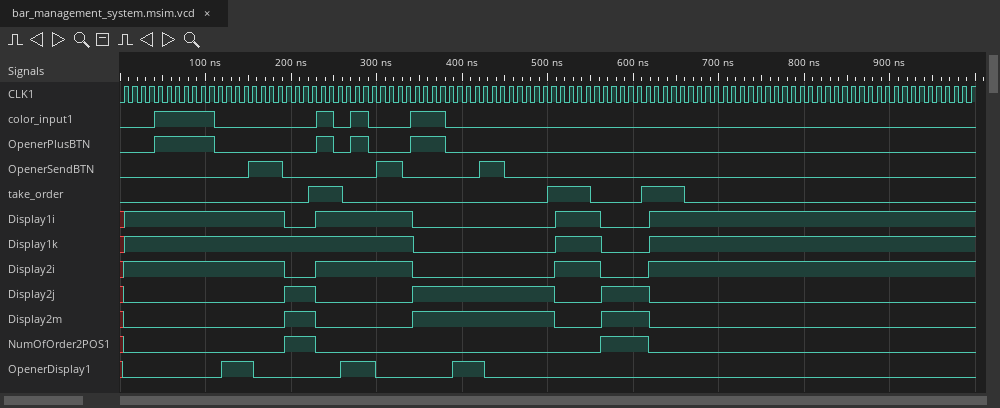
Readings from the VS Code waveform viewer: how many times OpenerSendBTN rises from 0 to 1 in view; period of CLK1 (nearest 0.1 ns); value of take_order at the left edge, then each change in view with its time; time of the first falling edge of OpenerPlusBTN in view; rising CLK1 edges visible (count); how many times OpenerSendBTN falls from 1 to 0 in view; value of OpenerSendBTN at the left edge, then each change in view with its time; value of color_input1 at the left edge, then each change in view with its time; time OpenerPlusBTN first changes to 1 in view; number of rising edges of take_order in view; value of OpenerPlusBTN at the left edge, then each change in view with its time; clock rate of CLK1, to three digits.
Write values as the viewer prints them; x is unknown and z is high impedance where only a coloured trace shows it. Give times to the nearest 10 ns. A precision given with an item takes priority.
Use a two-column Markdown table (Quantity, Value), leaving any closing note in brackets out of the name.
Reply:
| Quantity | Value |
|---|---|
| how many times OpenerSendBTN rises from 0 to 1 in view | 3 |
| period of CLK1 | 10 ns |
| value of take_order at the left edge, then each change in view with its time | 0, 1 at 220 ns, 0 at 260 ns, 1 at 500 ns, 0 at 550 ns, 1 at 610 ns, 0 at 660 ns |
| time of the first falling edge of OpenerPlusBTN in view | 110 ns |
| rising CLK1 edges visible | 100 |
| how many times OpenerSendBTN falls from 1 to 0 in view | 3 |
| value of OpenerSendBTN at the left edge, then each change in view with its time | 0, 1 at 150 ns, 0 at 190 ns, 1 at 300 ns, 0 at 330 ns, 1 at 420 ns, 0 at 450 ns |
| value of color_input1 at the left edge, then each change in view with its time | 0, 1 at 40 ns, 0 at 110 ns, 1 at 230 ns, 0 at 250 ns, 1 at 270 ns, 0 at 290 ns, 1 at 340 ns, 0 at 380 ns |
| time OpenerPlusBTN first changes to 1 in view | 40 ns |
| number of rising edges of take_order in view | 3 |
| value of OpenerPlusBTN at the left edge, then each change in view with its time | 0, 1 at 40 ns, 0 at 110 ns, 1 at 230 ns, 0 at 250 ns, 1 at 270 ns, 0 at 290 ns, 1 at 340 ns, 0 at 380 ns |
| clock rate of CLK1, to three digits | 100 MHz |
